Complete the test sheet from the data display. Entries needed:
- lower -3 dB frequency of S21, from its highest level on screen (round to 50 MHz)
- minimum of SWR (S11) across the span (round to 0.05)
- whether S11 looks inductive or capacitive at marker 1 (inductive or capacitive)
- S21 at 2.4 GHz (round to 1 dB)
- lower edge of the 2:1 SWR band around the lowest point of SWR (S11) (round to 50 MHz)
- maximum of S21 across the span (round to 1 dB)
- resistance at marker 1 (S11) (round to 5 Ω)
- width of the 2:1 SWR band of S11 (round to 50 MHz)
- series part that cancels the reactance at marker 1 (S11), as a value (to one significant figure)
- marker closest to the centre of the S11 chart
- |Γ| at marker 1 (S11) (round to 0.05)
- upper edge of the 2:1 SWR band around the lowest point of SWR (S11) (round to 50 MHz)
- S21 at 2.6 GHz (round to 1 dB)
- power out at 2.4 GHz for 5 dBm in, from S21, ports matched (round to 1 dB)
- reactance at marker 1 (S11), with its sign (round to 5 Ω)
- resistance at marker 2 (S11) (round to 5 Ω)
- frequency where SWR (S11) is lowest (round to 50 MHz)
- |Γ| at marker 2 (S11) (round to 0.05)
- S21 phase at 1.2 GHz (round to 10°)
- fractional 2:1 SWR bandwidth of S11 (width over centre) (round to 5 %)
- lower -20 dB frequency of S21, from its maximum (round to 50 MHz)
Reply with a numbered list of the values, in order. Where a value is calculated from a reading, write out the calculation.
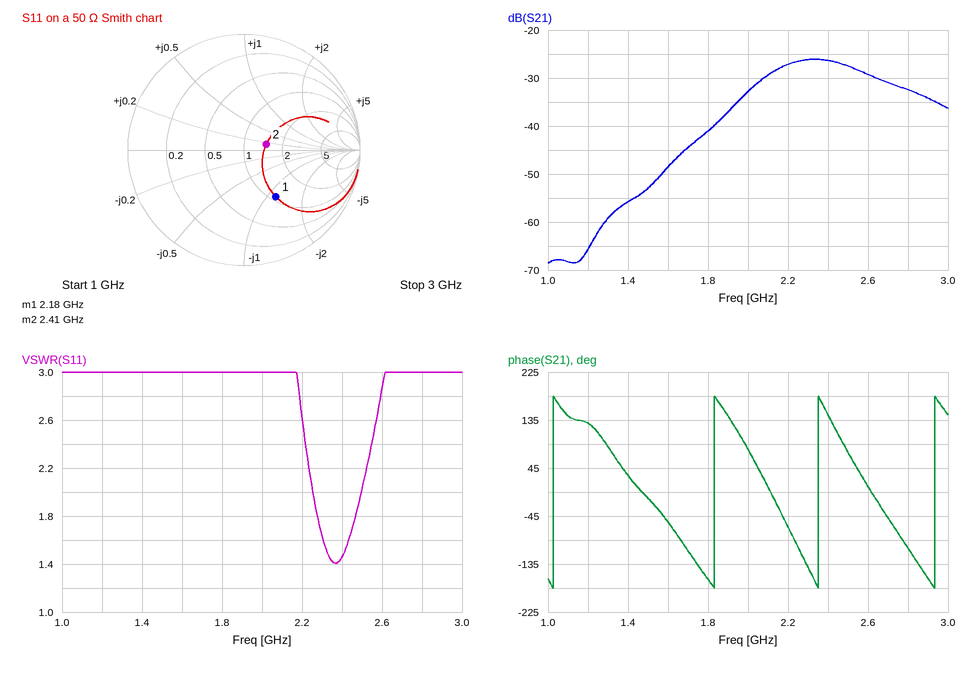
1. 2.10 GHz
2. 1.40
3. capacitive
4. -26 dB
5. 2.25 GHz
6. -26 dB
7. 55 Ω
8. 2.50 GHz − 2.25 GHz = 250 MHz
9. L = 60 Ω/(2π × 2.18 GHz) ≈ 4 nH
10. marker 2
11. 0.50
12. 2.50 GHz
13. -29 dB
14. 5 dBm + (-26 dB) = -21 dBm
15. -60 Ω
16. 75 Ω
17. 2.35 GHz
18. 0.20
19. 130°
20. 250 MHz / 2.375 GHz ≈ 10 %
21. 1.65 GHz
